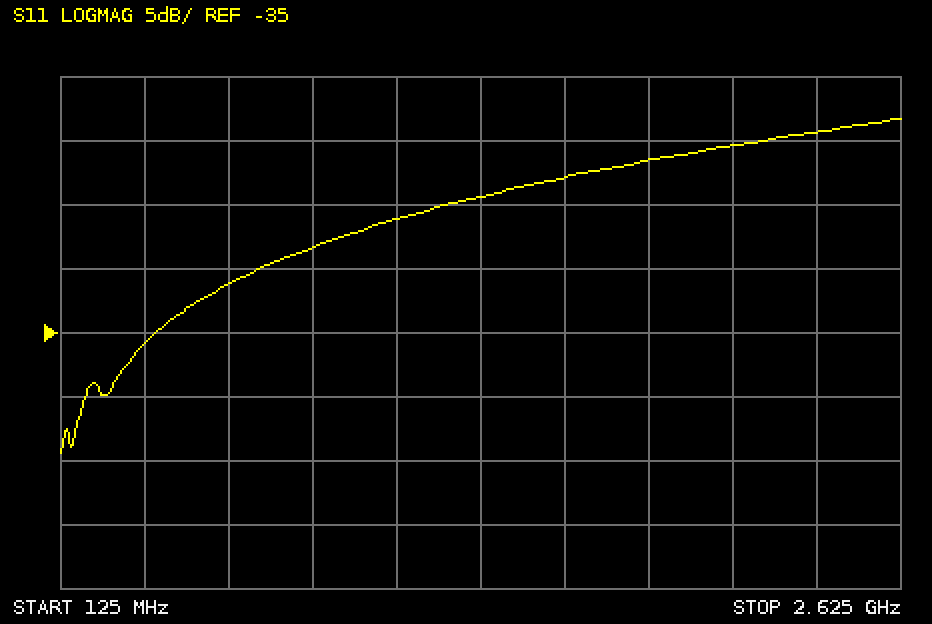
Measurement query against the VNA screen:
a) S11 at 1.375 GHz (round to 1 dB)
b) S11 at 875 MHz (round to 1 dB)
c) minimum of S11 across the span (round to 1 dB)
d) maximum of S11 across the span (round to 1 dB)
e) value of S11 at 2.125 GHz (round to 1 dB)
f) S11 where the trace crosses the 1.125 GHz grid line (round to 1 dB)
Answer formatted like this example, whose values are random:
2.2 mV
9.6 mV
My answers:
-24 dB
-28 dB
-44 dB
-18 dB
-20 dB
-26 dB
